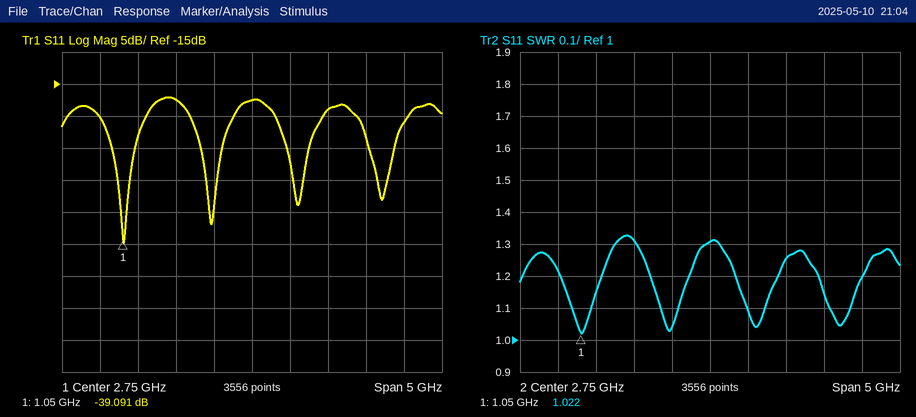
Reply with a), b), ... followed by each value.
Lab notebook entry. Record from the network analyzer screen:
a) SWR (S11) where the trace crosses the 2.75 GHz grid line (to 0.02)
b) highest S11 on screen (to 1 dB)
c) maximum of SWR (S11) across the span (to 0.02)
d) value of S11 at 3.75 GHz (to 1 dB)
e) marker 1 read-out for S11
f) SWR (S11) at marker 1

a) 1.30
b) -17 dB
c) 1.32
d) -19 dB
e) -39.091 dB
f) 1.022
